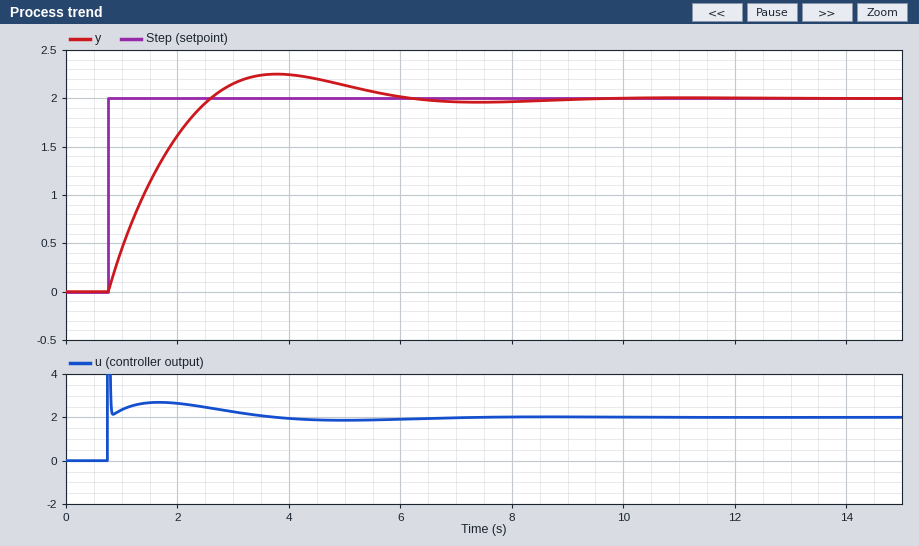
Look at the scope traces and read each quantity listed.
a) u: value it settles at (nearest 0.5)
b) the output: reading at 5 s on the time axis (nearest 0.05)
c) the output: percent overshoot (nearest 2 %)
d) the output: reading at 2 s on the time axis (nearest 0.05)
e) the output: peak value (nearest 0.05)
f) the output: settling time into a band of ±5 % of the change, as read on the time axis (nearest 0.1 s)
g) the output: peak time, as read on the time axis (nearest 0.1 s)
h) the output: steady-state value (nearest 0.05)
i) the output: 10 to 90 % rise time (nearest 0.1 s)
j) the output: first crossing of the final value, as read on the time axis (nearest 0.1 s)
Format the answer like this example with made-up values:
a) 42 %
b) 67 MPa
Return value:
a) 2.0
b) 2.15
c) 12 %
d) 1.60
e) 2.25
f) 5.3 s
g) 3.8 s
h) 2.00
i) 1.4 s
j) 2.6 s
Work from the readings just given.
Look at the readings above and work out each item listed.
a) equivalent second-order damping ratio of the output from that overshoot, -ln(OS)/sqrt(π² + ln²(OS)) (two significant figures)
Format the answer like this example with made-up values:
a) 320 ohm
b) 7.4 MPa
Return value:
a) 0.56
